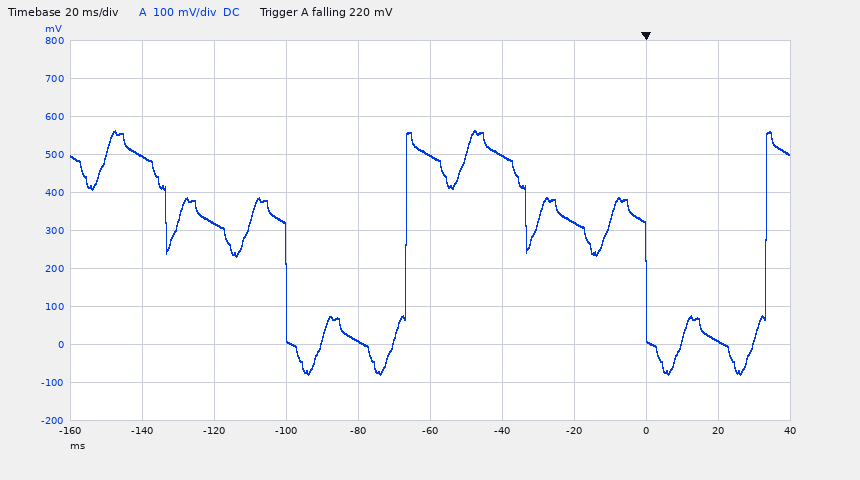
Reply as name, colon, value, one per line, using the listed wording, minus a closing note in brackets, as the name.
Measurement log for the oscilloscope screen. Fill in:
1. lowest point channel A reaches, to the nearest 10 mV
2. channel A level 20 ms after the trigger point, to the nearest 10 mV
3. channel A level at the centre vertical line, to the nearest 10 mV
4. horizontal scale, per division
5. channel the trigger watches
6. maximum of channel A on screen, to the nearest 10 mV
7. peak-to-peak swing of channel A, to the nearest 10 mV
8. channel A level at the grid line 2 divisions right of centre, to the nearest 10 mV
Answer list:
lowest point channel A reaches, to the nearest 10 mV: -80 mV
channel A level 20 ms after the trigger point, to the nearest 10 mV: 10 mV
channel A level at the centre vertical line, to the nearest 10 mV: 500 mV
horizontal scale, per division: 20 ms
channel the trigger watches: channel A
maximum of channel A on screen, to the nearest 10 mV: 560 mV
peak-to-peak swing of channel A, to the nearest 10 mV: 640 mV
channel A level at the grid line 2 divisions right of centre, to the nearest 10 mV: 320 mV
